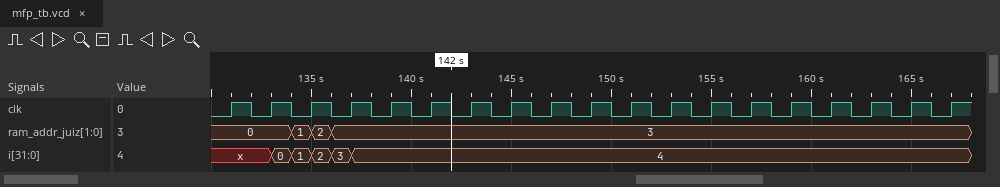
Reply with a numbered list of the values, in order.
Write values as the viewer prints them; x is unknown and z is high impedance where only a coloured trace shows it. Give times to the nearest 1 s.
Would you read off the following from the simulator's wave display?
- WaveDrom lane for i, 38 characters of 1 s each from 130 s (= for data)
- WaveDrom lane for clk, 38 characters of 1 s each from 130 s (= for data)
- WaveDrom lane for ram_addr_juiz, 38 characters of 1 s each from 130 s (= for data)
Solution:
1. {name: 'i', wave: 'x..=====..............................', data: '0 1 2 3 4'}
2. {name: 'clk', wave: '01010101010101010101010101010101010101'}
3. {name: 'ram_addr_juiz', wave: '=...===...............................', data: '0 1 2 3'}
